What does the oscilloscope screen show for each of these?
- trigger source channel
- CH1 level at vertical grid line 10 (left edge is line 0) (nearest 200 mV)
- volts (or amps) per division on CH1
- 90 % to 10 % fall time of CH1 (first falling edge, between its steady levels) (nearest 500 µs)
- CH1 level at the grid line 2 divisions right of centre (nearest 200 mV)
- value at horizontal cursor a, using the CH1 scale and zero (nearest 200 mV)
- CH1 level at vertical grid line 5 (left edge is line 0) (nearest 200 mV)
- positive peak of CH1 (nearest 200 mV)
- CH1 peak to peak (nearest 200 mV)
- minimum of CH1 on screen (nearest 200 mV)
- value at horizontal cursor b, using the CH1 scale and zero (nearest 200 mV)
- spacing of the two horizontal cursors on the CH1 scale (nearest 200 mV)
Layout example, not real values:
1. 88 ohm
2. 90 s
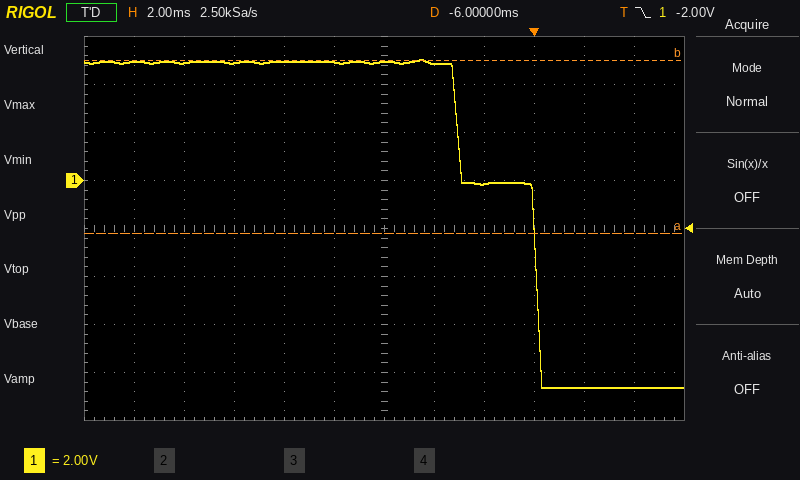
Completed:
1. CH1
2. -8.6 V
3. 2 V
4. 3.5 ms
5. -200 mV
6. -2.2 V
7. 5.0 V
8. 5.0 V
9. 13.6 V
10. -8.6 V
11. 5.0 V
12. 7.2 V
